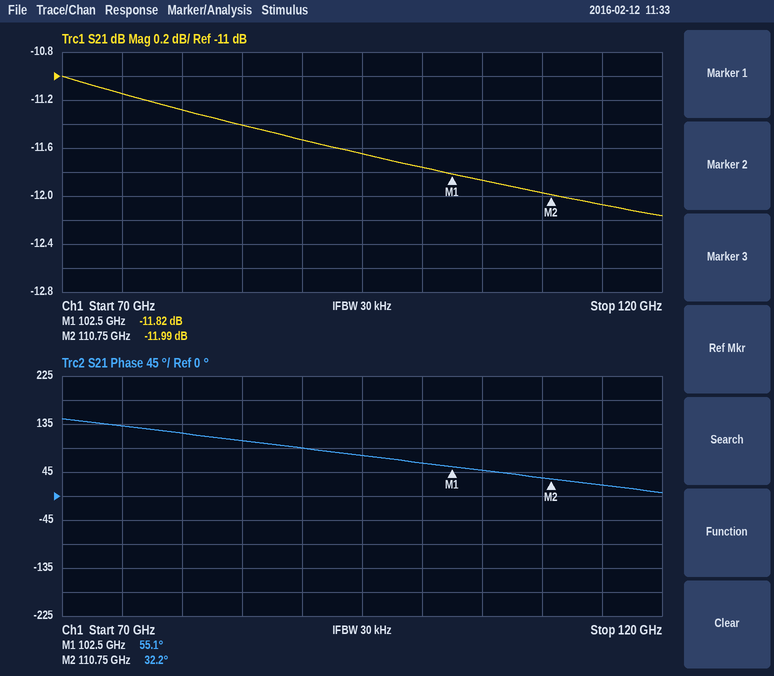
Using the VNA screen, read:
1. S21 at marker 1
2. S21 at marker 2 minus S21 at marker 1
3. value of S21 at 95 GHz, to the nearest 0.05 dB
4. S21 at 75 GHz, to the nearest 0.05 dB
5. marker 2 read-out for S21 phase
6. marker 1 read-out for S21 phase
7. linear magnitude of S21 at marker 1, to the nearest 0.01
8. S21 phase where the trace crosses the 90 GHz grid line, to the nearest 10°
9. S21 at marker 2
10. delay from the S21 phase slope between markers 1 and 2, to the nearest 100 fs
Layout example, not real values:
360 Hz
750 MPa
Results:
-11.82 dB
-0.17 dB
-11.65 dB
-11.15 dB
32.2°
55.1°
0.26
90°
-11.99 dB
7.7 ps
